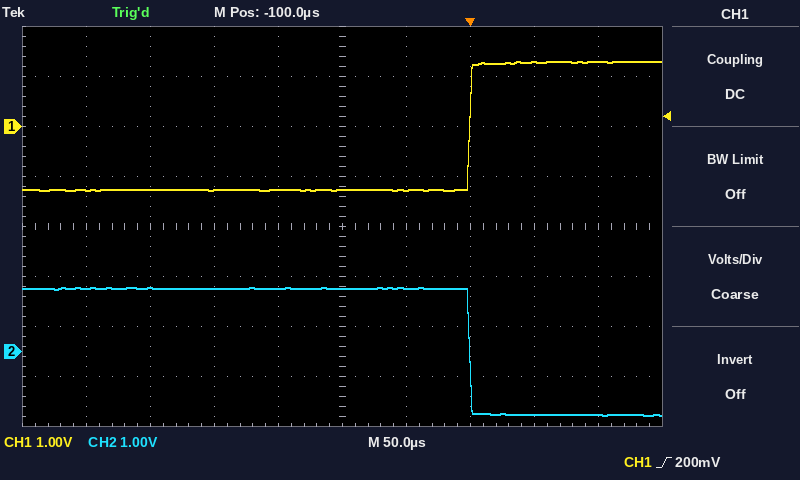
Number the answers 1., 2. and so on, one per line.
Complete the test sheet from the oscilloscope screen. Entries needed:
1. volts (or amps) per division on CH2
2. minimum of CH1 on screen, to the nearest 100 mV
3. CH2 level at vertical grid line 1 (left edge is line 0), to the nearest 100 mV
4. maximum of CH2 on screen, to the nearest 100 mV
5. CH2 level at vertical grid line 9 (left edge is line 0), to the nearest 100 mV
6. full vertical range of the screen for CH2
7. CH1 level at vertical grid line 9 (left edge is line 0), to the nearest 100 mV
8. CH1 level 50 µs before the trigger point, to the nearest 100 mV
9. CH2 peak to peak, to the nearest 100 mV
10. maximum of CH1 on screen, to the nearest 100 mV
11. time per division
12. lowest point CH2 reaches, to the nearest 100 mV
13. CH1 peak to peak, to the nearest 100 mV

1. 1 V
2. -1.3 V
3. 1.3 V
4. 1.3 V
5. -1.3 V
6. 8 V
7. 1.3 V
8. -1.3 V
9. 2.6 V
10. 1.3 V
11. 50 µs
12. -1.3 V
13. 2.6 V
